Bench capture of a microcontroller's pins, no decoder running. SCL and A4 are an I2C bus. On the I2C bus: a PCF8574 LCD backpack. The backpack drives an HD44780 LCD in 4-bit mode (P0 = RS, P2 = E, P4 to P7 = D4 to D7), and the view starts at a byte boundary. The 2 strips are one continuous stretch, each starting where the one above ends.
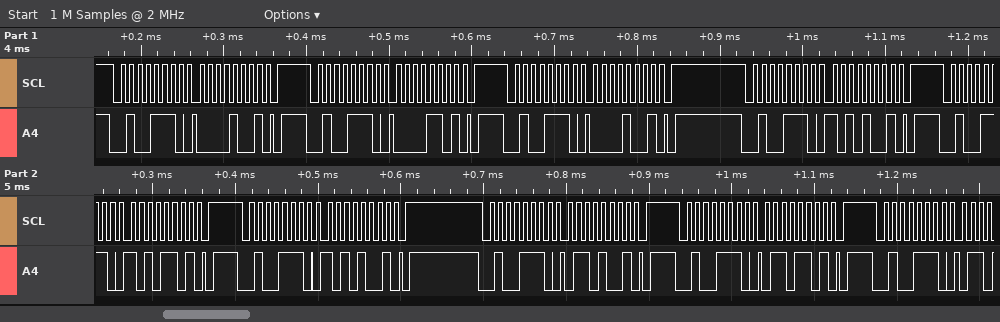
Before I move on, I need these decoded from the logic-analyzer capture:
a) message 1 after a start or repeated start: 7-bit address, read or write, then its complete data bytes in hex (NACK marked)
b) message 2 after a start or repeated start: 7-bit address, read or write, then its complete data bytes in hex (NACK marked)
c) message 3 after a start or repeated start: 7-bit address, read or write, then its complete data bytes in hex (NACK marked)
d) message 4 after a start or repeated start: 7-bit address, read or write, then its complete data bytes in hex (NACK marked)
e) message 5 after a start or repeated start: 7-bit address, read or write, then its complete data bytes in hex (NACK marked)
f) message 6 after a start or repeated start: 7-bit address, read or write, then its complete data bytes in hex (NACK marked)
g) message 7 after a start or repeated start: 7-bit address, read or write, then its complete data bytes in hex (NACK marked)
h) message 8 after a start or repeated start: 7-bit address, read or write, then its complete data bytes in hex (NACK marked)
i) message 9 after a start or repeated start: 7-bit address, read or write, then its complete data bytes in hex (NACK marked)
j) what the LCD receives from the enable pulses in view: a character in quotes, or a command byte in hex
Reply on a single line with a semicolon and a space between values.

0x27 write: 09; 0x27 write: 0D; 0x27 write: 09; 0x27 write: A9; 0x27 write: AD; 0x27 write: A9; 0x27 write: 69; 0x27 write: 6D; 0x27 write; data 0x0A
